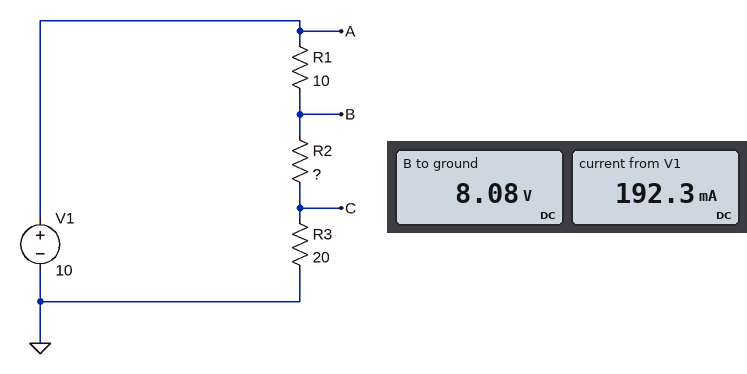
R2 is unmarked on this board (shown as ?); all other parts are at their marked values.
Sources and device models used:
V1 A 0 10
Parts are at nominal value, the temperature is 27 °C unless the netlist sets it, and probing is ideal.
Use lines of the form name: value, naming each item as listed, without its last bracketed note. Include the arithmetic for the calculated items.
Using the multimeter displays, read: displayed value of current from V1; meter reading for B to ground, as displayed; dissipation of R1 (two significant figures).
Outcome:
displayed value of current from V1: 192.3 mA
meter reading for B to ground, as displayed: 8.08 V
dissipation of R1: (10 V - 8.08 V)^2 / 10 Ω = 370 mW
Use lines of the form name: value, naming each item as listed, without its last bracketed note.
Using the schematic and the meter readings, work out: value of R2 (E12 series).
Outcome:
value of R2: 22 Ω
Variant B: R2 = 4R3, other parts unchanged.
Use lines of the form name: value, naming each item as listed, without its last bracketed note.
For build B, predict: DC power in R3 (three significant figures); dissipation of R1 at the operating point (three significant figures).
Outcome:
DC power in R3: 1.70 W
dissipation of R1 at the operating point: 850 mW
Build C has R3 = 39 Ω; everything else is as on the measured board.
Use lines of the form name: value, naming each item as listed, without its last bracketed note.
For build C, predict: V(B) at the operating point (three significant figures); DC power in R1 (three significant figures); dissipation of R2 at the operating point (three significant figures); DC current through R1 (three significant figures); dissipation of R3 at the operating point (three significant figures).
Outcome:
V(B) at the operating point: 8.59 V
DC power in R1: 198 mW
dissipation of R2 at the operating point: 436 mW
DC current through R1: 141 mA
dissipation of R3 at the operating point: 774 mW
